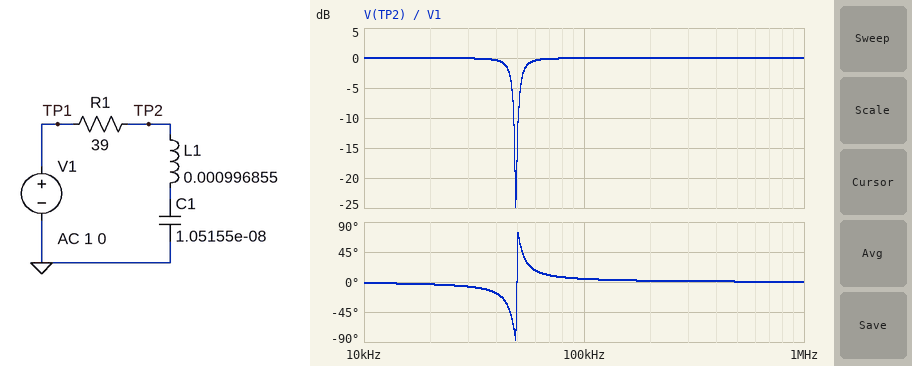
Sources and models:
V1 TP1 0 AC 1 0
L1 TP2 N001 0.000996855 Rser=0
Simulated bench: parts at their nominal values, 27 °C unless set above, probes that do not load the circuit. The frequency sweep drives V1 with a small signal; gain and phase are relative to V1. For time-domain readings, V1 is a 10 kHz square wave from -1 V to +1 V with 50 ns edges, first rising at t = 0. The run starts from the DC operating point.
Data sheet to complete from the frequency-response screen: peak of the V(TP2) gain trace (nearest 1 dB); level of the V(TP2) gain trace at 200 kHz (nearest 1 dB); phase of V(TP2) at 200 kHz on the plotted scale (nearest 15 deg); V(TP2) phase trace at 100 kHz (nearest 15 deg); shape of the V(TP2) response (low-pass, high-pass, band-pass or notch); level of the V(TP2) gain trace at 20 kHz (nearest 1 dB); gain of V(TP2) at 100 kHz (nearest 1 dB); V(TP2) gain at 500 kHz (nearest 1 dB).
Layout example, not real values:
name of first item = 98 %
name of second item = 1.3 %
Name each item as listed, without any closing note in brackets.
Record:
peak of the V(TP2) gain trace = 0 dB
level of the V(TP2) gain trace at 200 kHz = 0 dB
phase of V(TP2) at 200 kHz on the plotted scale = 0 deg
V(TP2) phase trace at 100 kHz = 0 deg
shape of the V(TP2) response = notch
level of the V(TP2) gain trace at 20 kHz = 0 dB
gain of V(TP2) at 100 kHz = 0 dB
V(TP2) gain at 500 kHz = 0 dB
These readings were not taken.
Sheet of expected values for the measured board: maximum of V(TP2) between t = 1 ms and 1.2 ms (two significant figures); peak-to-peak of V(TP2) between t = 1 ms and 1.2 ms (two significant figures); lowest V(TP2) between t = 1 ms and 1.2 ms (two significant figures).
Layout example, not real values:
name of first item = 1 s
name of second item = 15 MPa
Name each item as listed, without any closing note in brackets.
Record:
maximum of V(TP2) between t = 1 ms and 1.2 ms = 1.3 V
peak-to-peak of V(TP2) between t = 1 ms and 1.2 ms = 2.6 V
lowest V(TP2) between t = 1 ms and 1.2 ms = -1.3 V
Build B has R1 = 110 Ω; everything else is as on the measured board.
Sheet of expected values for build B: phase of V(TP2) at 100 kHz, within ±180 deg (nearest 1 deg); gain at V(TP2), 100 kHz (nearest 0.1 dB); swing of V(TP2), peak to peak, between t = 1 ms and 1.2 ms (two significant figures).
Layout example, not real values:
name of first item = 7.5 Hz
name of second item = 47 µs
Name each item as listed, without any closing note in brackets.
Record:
phase of V(TP2) at 100 kHz, within ±180 deg = 13 deg
gain at V(TP2), 100 kHz = -0.2 dB
swing of V(TP2), peak to peak, between t = 1 ms and 1.2 ms = 2.7 V
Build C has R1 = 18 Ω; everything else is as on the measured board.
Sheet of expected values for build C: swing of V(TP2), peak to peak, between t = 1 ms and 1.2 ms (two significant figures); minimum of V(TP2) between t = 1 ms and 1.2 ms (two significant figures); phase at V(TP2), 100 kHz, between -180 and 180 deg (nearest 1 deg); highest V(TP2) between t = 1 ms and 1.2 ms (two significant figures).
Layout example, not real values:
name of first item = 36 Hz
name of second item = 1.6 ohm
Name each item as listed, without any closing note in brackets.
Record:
swing of V(TP2), peak to peak, between t = 1 ms and 1.2 ms = 2.5 V
minimum of V(TP2) between t = 1 ms and 1.2 ms = -1.2 V
phase at V(TP2), 100 kHz, between -180 and 180 deg = 2 deg
highest V(TP2) between t = 1 ms and 1.2 ms = 1.2 V
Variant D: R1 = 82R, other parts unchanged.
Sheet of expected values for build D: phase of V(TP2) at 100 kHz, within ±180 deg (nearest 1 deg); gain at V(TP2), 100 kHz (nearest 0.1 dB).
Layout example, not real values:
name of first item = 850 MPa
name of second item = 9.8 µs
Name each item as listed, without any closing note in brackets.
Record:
phase of V(TP2) at 100 kHz, within ±180 deg = 10 deg
gain at V(TP2), 100 kHz = -0.1 dB
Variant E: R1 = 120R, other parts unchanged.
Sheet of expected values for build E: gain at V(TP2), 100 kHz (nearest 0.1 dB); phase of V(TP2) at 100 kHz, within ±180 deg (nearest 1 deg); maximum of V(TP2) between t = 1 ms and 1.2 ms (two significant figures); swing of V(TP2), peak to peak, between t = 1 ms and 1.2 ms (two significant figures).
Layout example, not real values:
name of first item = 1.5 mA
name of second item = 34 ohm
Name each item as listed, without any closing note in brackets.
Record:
gain at V(TP2), 100 kHz = -0.3 dB
phase of V(TP2) at 100 kHz, within ±180 deg = 14 deg
maximum of V(TP2) between t = 1 ms and 1.2 ms = 1.3 V
swing of V(TP2), peak to peak, between t = 1 ms and 1.2 ms = 2.7 V
